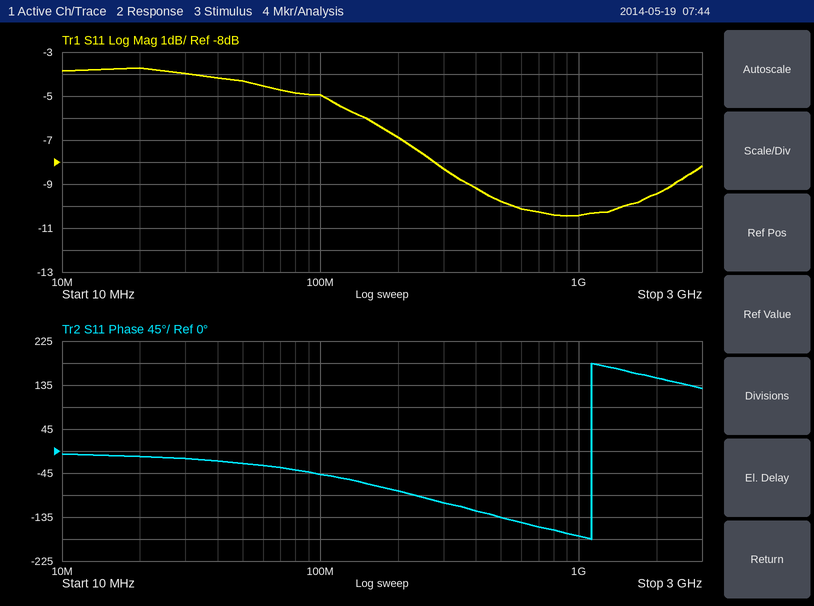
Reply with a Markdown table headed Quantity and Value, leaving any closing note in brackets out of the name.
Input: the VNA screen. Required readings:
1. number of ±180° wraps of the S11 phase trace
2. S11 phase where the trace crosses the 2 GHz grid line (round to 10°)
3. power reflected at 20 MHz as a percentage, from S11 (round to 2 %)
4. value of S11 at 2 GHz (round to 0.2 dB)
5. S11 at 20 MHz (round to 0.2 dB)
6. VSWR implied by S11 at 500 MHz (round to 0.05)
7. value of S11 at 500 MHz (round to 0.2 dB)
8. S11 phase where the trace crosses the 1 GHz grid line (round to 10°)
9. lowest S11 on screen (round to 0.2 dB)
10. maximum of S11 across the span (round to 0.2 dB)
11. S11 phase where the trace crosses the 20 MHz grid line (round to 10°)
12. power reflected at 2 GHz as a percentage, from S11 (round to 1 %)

| Quantity | Value |
|---|---|
| number of ±180° wraps of the S11 phase trace | 1 |
| S11 phase where the trace crosses the 2 GHz grid line | 150° |
| power reflected at 20 MHz as a percentage, from S11 | 42 % |
| value of S11 at 2 GHz | -9.4 dB |
| S11 at 20 MHz | -3.8 dB |
| VSWR implied by S11 at 500 MHz | 1.95 |
| value of S11 at 500 MHz | -9.8 dB |
| S11 phase where the trace crosses the 1 GHz grid line | -170° |
| lowest S11 on screen | -10.4 dB |
| maximum of S11 across the span | -3.8 dB |
| S11 phase where the trace crosses the 20 MHz grid line | -10° |
| power reflected at 2 GHz as a percentage, from S11 | 11 % |
